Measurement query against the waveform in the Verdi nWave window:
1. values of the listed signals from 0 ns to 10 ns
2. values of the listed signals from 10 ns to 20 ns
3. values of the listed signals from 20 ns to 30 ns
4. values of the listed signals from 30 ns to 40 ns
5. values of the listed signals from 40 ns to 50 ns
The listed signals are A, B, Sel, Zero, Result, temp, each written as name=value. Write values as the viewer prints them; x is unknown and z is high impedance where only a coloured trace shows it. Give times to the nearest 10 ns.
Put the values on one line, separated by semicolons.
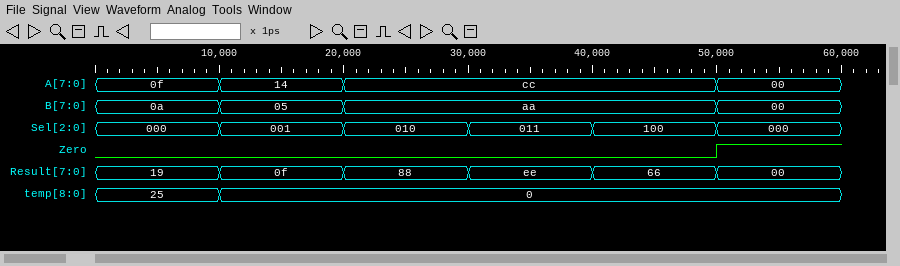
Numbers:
A=0f, B=0a, Sel=000, Zero=0, Result=19, temp=25; A=14, B=05, Sel=001, Zero=0, Result=0f, temp=0; A=cc, B=aa, Sel=010, Zero=0, Result=88, temp=0; A=cc, B=aa, Sel=011, Zero=0, Result=ee, temp=0; A=cc, B=aa, Sel=100, Zero=0, Result=66, temp=0
